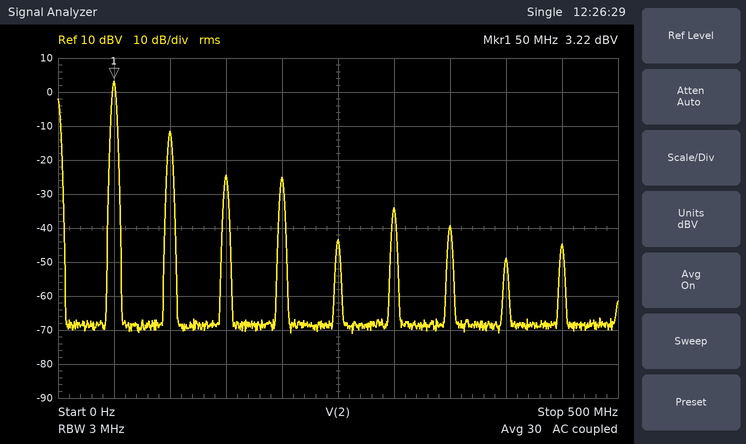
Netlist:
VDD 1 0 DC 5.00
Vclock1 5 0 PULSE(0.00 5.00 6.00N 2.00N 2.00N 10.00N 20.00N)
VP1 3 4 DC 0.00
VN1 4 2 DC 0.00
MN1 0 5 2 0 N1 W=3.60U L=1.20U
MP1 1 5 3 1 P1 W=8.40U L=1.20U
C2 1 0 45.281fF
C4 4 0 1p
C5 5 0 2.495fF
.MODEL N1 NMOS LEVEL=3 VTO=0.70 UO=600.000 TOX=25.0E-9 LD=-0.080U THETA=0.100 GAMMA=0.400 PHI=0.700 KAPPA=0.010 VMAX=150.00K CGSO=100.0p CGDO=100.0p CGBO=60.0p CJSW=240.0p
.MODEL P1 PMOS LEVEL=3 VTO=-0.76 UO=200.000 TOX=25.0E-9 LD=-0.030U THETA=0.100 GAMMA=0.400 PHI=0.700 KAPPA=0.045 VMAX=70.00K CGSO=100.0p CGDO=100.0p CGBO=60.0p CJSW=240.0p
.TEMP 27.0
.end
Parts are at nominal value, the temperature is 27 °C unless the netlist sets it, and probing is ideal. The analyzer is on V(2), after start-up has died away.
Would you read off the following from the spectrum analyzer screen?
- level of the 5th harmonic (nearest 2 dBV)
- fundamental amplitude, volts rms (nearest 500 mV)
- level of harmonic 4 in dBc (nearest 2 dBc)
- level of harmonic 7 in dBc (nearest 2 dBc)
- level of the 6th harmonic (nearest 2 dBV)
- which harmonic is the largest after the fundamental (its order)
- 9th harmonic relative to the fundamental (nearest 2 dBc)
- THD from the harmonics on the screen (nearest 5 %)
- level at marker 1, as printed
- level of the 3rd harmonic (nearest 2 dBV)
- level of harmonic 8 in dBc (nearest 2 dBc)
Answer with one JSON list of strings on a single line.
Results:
["-44 dBV", "1.5 V", "-28 dBc", "-42 dBc", "-34 dBV", "2", "-48 dBc", "20 %", "3.22 dBV", "-24 dBV", "-52 dBc"]
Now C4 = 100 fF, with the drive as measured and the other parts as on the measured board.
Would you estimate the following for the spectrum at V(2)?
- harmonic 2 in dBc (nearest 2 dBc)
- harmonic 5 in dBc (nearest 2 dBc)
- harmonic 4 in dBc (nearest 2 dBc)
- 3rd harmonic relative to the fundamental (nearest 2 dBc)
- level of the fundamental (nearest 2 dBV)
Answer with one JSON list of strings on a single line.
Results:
["-10 dBc", "-38 dBc", "-12 dBc", "-14 dBc", "6 dBV"]
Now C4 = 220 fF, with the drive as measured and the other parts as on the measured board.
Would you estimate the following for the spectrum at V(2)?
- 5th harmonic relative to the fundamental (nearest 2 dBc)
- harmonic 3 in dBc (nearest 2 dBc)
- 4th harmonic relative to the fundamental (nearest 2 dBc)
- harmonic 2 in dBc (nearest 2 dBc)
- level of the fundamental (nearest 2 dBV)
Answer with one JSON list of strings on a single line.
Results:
["-38 dBc", "-16 dBc", "-14 dBc", "-10 dBc", "6 dBV"]
